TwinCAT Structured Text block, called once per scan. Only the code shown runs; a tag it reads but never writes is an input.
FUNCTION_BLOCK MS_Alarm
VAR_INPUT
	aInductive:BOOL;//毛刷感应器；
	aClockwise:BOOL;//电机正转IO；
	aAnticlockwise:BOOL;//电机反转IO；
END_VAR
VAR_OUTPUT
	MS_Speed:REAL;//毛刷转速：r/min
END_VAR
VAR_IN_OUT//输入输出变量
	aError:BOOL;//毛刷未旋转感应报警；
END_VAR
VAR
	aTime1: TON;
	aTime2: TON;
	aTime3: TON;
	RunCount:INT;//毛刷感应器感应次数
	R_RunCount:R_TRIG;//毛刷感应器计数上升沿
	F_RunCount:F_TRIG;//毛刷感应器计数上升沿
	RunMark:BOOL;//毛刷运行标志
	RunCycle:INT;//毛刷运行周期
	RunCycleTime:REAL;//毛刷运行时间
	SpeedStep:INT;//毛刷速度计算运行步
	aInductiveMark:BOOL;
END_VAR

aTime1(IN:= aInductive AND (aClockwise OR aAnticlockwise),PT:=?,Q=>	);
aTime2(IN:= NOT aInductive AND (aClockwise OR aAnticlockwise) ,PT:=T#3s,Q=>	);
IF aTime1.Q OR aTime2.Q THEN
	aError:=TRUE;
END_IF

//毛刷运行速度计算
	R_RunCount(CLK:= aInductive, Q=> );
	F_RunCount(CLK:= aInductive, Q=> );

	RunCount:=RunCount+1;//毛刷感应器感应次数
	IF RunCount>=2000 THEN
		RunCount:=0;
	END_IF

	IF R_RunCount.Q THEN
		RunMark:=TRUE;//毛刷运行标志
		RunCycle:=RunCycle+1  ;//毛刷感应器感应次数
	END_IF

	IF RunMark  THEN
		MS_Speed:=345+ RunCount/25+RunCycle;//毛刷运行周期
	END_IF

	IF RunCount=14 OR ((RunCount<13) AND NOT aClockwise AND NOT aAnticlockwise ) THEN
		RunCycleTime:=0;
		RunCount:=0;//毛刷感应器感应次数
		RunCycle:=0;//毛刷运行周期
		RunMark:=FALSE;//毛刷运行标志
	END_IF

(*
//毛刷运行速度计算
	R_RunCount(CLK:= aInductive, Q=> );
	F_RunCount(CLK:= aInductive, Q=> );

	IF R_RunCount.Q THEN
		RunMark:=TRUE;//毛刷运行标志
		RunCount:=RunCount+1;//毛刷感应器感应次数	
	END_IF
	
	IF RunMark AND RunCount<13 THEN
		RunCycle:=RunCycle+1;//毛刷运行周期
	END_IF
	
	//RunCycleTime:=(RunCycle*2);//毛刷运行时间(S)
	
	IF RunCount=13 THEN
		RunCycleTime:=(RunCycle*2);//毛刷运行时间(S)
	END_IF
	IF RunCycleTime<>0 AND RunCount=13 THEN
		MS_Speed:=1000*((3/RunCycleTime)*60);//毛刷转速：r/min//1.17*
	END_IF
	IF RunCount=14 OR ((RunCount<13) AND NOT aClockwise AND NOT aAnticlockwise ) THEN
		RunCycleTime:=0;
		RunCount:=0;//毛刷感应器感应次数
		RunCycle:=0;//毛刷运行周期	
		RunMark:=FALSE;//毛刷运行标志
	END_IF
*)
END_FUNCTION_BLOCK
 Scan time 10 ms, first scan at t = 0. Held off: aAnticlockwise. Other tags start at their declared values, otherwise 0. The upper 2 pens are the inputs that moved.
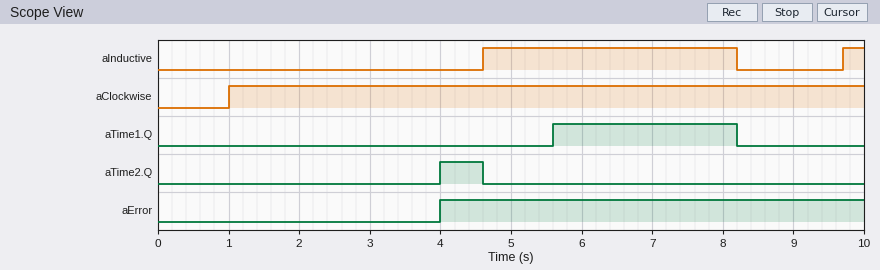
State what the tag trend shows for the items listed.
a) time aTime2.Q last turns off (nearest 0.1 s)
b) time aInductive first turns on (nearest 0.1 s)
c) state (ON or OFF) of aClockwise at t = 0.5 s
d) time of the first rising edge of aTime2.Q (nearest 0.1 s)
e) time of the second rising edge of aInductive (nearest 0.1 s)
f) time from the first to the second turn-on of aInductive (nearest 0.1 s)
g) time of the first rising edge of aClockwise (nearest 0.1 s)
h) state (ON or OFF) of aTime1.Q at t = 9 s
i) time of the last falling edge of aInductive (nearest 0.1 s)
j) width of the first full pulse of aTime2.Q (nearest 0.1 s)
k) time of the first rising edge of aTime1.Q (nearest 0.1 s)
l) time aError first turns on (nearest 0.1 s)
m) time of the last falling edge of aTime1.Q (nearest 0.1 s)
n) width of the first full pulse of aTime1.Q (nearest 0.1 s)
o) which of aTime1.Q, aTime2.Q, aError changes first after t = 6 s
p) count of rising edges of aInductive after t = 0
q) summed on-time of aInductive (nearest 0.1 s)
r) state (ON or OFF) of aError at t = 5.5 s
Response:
4.6 s
4.6 s
OFF
4.0 s
9.7 s
5.1 s
1.0 s
OFF
8.2 s
0.6 s
5.6 s
4.0 s
8.2 s
2.6 s
aTime1.Q
2
3.9 s
ON
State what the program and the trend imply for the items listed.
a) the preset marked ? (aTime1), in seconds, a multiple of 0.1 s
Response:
1.0 s
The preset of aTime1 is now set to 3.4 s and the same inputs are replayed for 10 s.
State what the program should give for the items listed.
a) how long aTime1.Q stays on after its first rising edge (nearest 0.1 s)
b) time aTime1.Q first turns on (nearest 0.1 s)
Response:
0.2 s
8.0 s
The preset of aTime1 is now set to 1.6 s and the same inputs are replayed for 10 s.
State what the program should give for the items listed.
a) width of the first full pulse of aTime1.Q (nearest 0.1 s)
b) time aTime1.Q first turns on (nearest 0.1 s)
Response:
2.0 s
6.2 s
